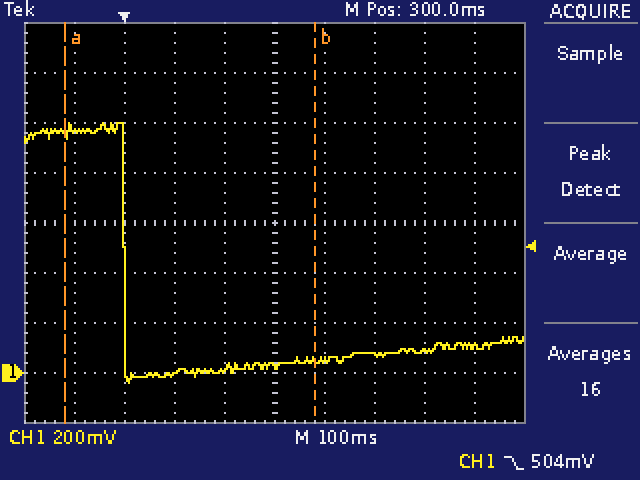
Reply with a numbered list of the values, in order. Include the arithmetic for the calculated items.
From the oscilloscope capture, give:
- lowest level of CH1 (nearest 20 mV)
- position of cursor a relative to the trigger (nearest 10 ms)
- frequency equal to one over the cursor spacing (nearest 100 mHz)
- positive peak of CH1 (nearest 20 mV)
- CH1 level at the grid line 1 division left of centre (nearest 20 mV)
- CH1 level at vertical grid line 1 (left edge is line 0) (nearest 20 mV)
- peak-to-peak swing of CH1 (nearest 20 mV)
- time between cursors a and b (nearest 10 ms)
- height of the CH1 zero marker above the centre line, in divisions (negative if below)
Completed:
1. -40 mV
2. -120 ms
3. 1 / 500 ms ≈ 2.0 Hz
4. 1.00 V
5. 20 mV
6. 980 mV
7. 1.00 V − (-40 mV) = 1.04 V
8. 500 ms
9. -3.0 div
